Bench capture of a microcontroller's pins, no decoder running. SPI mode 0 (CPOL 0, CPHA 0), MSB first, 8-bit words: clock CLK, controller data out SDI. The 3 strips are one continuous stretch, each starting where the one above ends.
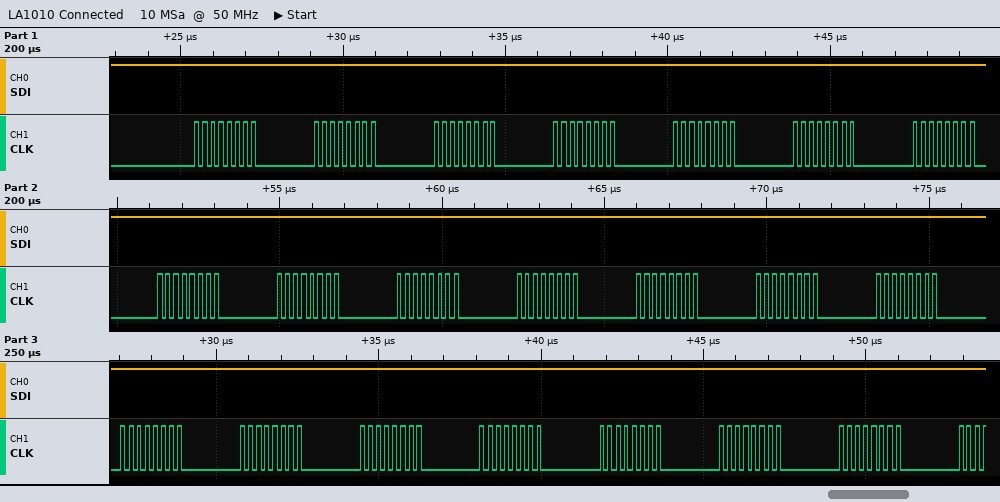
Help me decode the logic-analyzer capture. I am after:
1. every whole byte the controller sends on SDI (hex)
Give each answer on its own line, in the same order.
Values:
FF FF FF FF FF FF FF FF FF FF FF FF FF FF FF FF FF FF FF FF FF
